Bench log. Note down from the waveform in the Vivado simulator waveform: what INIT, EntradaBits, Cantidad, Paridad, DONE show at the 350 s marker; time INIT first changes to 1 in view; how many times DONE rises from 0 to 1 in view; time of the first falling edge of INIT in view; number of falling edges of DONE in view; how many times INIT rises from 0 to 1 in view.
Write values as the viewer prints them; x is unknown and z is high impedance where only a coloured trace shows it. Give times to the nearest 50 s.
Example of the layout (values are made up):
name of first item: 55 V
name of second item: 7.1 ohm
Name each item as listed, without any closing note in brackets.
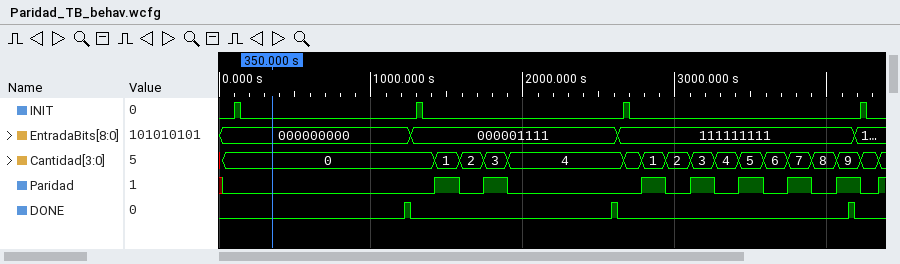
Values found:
what INIT, EntradaBits, Cantidad, Paridad, DONE show at the 350 s marker: INIT=0, EntradaBits=000000000, Cantidad=0, Paridad=0, DONE=0
time INIT first changes to 1 in view: 100 s
how many times DONE rises from 0 to 1 in view: 3
time of the first falling edge of INIT in view: 150 s
number of falling edges of DONE in view: 3
how many times INIT rises from 0 to 1 in view: 4
